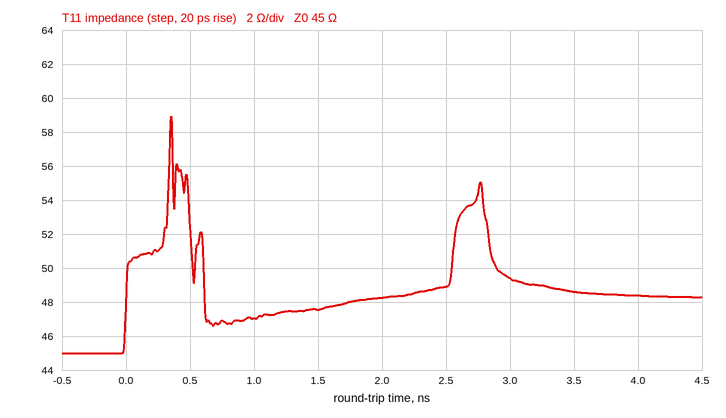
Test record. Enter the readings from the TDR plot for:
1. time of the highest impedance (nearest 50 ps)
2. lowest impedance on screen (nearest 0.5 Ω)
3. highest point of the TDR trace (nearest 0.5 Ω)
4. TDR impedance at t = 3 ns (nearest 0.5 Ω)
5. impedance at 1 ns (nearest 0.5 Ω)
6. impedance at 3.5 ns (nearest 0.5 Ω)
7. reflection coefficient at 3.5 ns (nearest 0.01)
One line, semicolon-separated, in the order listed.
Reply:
350 ps; 45.0 Ω; 59.0 Ω; 49.5 Ω; 47.0 Ω; 48.5 Ω; +0.04
